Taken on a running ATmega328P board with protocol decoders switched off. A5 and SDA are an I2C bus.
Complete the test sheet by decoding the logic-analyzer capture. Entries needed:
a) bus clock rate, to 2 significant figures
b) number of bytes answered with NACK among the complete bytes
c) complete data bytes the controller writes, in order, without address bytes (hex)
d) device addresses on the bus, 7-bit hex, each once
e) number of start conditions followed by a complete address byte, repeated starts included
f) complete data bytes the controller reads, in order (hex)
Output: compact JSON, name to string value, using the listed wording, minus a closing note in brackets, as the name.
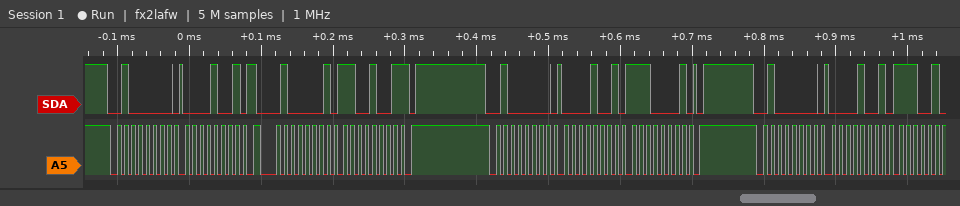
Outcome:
{"bus clock rate, to 2 significant figures": "100 kHz", "number of bytes answered with NACK among the complete bytes": "1", "complete data bytes the controller writes, in order, without address bytes": "09 09 E1 09", "device addresses on the bus, 7-bit hex, each once": "0x20", "number of start conditions followed by a complete address byte, repeated starts included": "4", "complete data bytes the controller reads, in order": "C9"}
